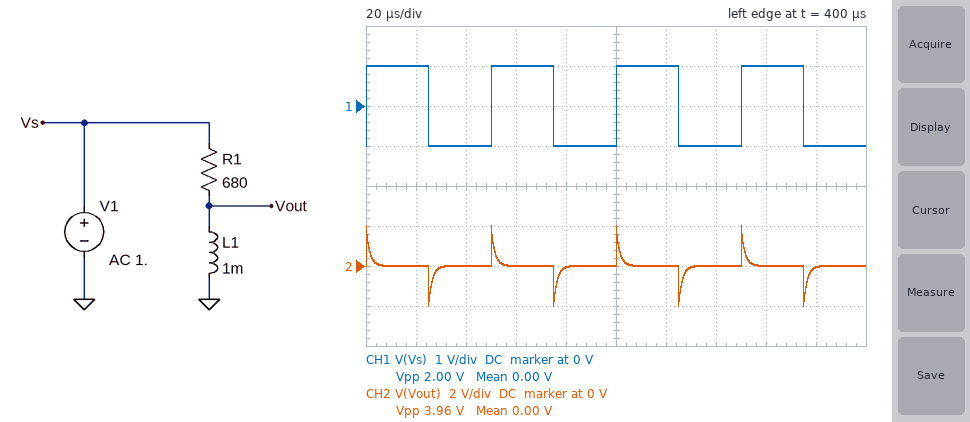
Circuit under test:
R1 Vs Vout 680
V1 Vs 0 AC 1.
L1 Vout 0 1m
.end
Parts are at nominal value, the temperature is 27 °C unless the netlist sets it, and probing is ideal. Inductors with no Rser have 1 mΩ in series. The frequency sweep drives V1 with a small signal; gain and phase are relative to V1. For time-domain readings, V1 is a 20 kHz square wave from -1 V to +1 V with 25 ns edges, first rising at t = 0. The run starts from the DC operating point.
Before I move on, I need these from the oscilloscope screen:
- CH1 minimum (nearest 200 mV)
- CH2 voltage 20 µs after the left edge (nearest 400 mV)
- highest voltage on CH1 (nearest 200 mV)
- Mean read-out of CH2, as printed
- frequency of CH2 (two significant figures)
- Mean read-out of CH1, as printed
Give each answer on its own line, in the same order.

-1.0 V
0 V
1.0 V
0.00 V
20 kHz
0.00 V
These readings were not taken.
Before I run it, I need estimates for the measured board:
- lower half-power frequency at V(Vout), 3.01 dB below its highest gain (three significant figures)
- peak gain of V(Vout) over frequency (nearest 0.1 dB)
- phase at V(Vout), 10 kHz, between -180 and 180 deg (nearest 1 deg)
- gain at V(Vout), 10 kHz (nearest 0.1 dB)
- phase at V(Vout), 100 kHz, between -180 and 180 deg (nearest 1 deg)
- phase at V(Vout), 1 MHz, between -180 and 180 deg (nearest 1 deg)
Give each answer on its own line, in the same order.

108 kHz
0 dB
85 deg
-20.7 dB
47 deg
6 deg
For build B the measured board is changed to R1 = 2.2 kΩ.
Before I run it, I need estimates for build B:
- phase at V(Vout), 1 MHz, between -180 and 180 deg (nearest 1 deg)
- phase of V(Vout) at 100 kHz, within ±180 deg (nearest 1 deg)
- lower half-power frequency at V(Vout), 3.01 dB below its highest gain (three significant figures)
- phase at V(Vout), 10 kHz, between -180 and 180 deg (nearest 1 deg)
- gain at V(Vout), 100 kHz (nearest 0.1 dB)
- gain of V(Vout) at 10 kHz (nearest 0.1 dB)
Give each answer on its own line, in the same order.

19 deg
74 deg
350 kHz
88 deg
-11.2 dB
-30.9 dB
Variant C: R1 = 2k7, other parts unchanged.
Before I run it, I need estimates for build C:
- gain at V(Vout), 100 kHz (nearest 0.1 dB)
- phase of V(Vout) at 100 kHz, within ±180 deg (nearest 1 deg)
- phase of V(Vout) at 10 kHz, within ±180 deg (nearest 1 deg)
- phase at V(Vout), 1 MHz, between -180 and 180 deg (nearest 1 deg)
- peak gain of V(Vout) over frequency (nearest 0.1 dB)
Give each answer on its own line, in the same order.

-12.9 dB
77 deg
89 deg
23 deg
0 dB
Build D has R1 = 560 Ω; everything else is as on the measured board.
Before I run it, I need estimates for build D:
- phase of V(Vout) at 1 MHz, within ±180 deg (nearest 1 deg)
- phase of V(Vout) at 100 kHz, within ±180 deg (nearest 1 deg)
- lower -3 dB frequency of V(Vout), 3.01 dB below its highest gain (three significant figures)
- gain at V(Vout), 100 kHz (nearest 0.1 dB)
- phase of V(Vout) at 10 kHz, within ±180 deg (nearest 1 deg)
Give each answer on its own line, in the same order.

5 deg
42 deg
89.1 kHz
-2.5 dB
84 deg
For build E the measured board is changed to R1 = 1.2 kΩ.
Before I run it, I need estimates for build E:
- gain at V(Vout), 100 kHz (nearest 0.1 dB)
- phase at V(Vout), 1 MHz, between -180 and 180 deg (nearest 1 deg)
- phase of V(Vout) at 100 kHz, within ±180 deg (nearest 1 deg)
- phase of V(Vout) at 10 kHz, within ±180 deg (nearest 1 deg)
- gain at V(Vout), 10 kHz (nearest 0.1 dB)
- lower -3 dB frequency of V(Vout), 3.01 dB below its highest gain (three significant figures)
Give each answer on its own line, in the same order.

-6.7 dB
11 deg
62 deg
87 deg
-25.6 dB
191 kHz
